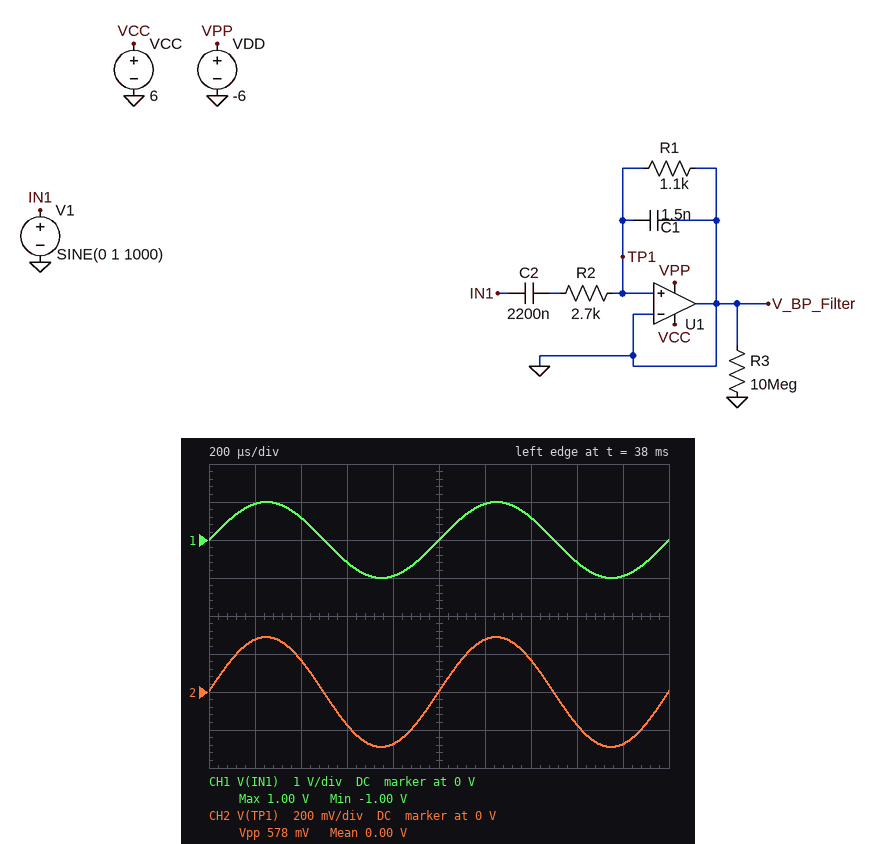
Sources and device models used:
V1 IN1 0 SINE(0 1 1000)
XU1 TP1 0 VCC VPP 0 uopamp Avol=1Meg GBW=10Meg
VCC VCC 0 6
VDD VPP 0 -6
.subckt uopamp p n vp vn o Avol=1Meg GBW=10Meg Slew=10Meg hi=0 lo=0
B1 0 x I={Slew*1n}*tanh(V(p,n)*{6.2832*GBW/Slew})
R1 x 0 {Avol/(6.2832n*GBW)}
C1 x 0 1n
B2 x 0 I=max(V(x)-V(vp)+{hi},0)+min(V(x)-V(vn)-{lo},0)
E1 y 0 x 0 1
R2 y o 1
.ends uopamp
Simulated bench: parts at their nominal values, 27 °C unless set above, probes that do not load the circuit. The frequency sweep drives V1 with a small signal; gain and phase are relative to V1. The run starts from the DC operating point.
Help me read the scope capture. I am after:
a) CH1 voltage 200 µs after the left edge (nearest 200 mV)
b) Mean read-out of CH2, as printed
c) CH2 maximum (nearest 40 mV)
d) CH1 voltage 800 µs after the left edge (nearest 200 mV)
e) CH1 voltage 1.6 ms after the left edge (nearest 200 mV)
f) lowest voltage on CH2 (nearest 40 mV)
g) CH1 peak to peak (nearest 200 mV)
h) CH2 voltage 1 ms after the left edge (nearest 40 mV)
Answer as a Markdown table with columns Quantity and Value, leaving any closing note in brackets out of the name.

| Quantity | Value |
|---|---|
| CH1 voltage 200 µs after the left edge | 1.0 V |
| Mean read-out of CH2, as printed | 0.00 V |
| CH2 maximum | 280 mV |
| CH1 voltage 800 µs after the left edge | -1.0 V |
| CH1 voltage 1.6 ms after the left edge | -600 mV |
| lowest voltage on CH2 | -280 mV |
| CH1 peak to peak | 2.0 V |
| CH2 voltage 1 ms after the left edge | 0 V |
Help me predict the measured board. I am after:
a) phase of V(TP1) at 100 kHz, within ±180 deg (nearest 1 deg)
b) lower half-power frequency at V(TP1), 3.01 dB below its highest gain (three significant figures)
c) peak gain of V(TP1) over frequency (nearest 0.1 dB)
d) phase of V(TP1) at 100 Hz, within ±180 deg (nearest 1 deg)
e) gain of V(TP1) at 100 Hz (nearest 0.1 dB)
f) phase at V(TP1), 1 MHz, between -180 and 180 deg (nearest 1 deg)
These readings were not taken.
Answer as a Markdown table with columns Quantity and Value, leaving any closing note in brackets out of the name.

| Quantity | Value |
|---|---|
| phase of V(TP1) at 100 kHz, within ±180 deg | -36 deg |
| lower half-power frequency at V(TP1), 3.01 dB below its highest gain | 19.0 Hz |
| peak gain of V(TP1) over frequency | -10.8 dB |
| phase of V(TP1) at 100 Hz, within ±180 deg | 11 deg |
| gain of V(TP1) at 100 Hz | -10.9 dB |
| phase at V(TP1), 1 MHz, between -180 and 180 deg | -82 deg |
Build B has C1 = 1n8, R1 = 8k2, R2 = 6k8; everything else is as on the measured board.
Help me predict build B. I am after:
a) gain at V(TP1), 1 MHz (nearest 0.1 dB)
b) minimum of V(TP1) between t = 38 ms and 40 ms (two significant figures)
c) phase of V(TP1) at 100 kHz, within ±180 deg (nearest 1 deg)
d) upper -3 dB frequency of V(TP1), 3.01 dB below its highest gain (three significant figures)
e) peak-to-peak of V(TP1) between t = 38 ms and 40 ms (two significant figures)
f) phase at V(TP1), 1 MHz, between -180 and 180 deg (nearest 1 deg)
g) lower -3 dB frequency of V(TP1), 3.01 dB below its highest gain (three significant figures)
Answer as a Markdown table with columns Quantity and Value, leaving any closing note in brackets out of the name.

| Quantity | Value |
|---|---|
| gain at V(TP1), 1 MHz | -37.7 dB |
| minimum of V(TP1) between t = 38 ms and 40 ms | -550 mV |
| phase of V(TP1) at 100 kHz, within ±180 deg | -77 deg |
| upper -3 dB frequency of V(TP1), 3.01 dB below its highest gain | 23.8 kHz |
| peak-to-peak of V(TP1) between t = 38 ms and 40 ms | 1.1 V |
| phase at V(TP1), 1 MHz, between -180 and 180 deg | -89 deg |
| lower -3 dB frequency of V(TP1), 3.01 dB below its highest gain | 4.82 Hz |
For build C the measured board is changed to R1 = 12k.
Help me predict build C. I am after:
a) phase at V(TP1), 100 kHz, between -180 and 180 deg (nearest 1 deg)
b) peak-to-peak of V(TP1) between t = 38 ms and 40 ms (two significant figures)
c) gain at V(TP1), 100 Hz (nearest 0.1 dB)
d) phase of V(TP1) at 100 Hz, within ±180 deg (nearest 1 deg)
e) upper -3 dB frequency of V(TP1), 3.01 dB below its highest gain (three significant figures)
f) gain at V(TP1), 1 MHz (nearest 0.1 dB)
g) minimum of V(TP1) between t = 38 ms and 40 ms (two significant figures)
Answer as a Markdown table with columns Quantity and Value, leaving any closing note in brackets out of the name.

| Quantity | Value |
|---|---|
| phase at V(TP1), 100 kHz, between -180 and 180 deg | -64 deg |
| peak-to-peak of V(TP1) between t = 38 ms and 40 ms | 1.6 V |
| gain at V(TP1), 100 Hz | -1.8 dB |
| phase of V(TP1) at 100 Hz, within ±180 deg | 3 deg |
| upper -3 dB frequency of V(TP1), 3.01 dB below its highest gain | 48.2 kHz |
| gain at V(TP1), 1 MHz | -28.1 dB |
| minimum of V(TP1) between t = 38 ms and 40 ms | -820 mV |
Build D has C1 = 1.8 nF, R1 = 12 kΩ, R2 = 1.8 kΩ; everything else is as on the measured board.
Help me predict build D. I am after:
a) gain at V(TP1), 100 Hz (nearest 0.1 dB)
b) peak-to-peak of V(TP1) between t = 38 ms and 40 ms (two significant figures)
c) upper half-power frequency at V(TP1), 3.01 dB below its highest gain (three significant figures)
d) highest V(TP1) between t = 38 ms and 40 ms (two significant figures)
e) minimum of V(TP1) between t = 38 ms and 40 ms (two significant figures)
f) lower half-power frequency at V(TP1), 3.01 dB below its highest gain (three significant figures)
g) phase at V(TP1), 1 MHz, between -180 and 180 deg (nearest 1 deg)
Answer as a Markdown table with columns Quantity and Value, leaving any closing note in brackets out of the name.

| Quantity | Value |
|---|---|
| gain at V(TP1), 100 Hz | -1.2 dB |
| peak-to-peak of V(TP1) between t = 38 ms and 40 ms | 1.7 V |
| upper half-power frequency at V(TP1), 3.01 dB below its highest gain | 56.5 kHz |
| highest V(TP1) between t = 38 ms and 40 ms | 870 mV |
| minimum of V(TP1) between t = 38 ms and 40 ms | -870 mV |
| lower half-power frequency at V(TP1), 3.01 dB below its highest gain | 5.24 Hz |
| phase at V(TP1), 1 MHz, between -180 and 180 deg | -87 deg |
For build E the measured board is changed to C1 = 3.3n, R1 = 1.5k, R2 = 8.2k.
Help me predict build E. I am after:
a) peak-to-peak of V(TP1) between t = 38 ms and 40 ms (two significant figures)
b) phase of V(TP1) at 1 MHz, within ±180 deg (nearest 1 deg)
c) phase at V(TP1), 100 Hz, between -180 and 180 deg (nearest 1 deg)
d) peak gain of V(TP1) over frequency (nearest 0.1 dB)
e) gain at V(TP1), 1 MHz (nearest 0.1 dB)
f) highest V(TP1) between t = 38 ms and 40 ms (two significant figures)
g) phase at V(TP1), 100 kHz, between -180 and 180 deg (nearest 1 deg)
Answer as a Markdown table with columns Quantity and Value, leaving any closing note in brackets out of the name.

| Quantity | Value |
|---|---|
| peak-to-peak of V(TP1) between t = 38 ms and 40 ms | 310 mV |
| phase of V(TP1) at 1 MHz, within ±180 deg | -88 deg |
| phase at V(TP1), 100 Hz, between -180 and 180 deg | 4 deg |
| peak gain of V(TP1) over frequency | -16.2 dB |
| gain at V(TP1), 1 MHz | -44.6 dB |
| highest V(TP1) between t = 38 ms and 40 ms | 150 mV |
| phase at V(TP1), 100 kHz, between -180 and 180 deg | -69 deg |
